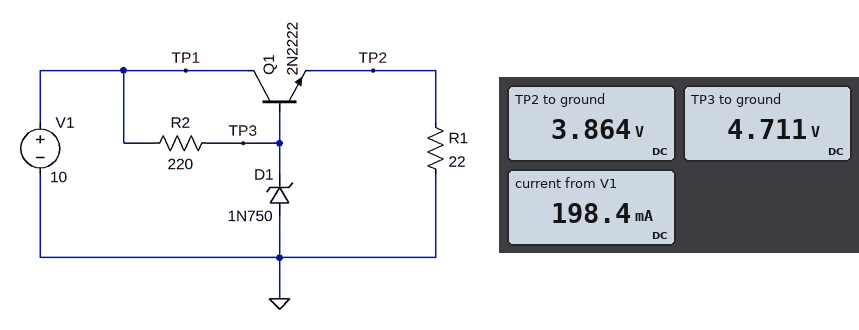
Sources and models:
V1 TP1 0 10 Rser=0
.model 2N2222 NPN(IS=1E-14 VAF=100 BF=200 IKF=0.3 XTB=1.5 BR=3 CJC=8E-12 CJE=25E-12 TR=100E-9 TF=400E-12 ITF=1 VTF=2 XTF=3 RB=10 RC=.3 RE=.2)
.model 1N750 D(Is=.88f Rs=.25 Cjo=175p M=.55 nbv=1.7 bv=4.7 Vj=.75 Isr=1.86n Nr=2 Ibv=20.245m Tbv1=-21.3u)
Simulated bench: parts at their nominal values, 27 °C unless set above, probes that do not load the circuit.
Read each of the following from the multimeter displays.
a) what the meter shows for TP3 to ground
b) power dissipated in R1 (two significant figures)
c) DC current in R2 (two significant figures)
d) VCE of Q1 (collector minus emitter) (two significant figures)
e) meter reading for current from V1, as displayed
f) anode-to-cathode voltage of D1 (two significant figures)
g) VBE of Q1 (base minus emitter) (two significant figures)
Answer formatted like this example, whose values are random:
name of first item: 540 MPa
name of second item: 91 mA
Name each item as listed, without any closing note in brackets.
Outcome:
what the meter shows for TP3 to ground: 4.711 V
power dissipated in R1: 680 mW
DC current in R2: 24 mA
VCE of Q1 (collector minus emitter): 6.1 V
meter reading for current from V1, as displayed: 198.4 mA
anode-to-cathode voltage of D1: -4.7 V
VBE of Q1 (base minus emitter): 850 mV
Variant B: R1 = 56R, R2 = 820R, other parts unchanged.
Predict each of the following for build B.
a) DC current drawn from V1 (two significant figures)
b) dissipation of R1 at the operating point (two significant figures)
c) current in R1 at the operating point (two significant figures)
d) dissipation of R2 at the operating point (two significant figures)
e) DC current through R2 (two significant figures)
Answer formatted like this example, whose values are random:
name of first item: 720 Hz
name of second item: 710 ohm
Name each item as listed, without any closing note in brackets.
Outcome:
DC current drawn from V1: 75 mA
dissipation of R1 at the operating point: 270 mW
current in R1 at the operating point: 69 mA
dissipation of R2 at the operating point: 35 mW
DC current through R2: 6.5 mA
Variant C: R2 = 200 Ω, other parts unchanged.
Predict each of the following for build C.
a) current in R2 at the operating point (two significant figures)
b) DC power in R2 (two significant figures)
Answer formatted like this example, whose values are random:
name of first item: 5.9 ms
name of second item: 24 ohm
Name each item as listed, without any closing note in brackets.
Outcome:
current in R2 at the operating point: 26 mA
DC power in R2: 140 mW
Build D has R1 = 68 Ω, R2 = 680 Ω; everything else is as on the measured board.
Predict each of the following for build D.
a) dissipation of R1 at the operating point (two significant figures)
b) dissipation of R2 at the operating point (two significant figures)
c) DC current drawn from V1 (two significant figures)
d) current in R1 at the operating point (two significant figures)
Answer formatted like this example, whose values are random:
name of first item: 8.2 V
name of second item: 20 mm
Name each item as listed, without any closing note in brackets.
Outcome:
dissipation of R1 at the operating point: 220 mW
dissipation of R2 at the operating point: 42 mW
DC current drawn from V1: 65 mA
current in R1 at the operating point: 57 mA
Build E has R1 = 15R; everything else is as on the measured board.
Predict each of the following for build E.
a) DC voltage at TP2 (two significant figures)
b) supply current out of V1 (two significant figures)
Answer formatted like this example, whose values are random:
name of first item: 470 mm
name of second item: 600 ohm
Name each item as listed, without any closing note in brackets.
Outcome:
DC voltage at TP2: 3.8 V
supply current out of V1: 280 mA
